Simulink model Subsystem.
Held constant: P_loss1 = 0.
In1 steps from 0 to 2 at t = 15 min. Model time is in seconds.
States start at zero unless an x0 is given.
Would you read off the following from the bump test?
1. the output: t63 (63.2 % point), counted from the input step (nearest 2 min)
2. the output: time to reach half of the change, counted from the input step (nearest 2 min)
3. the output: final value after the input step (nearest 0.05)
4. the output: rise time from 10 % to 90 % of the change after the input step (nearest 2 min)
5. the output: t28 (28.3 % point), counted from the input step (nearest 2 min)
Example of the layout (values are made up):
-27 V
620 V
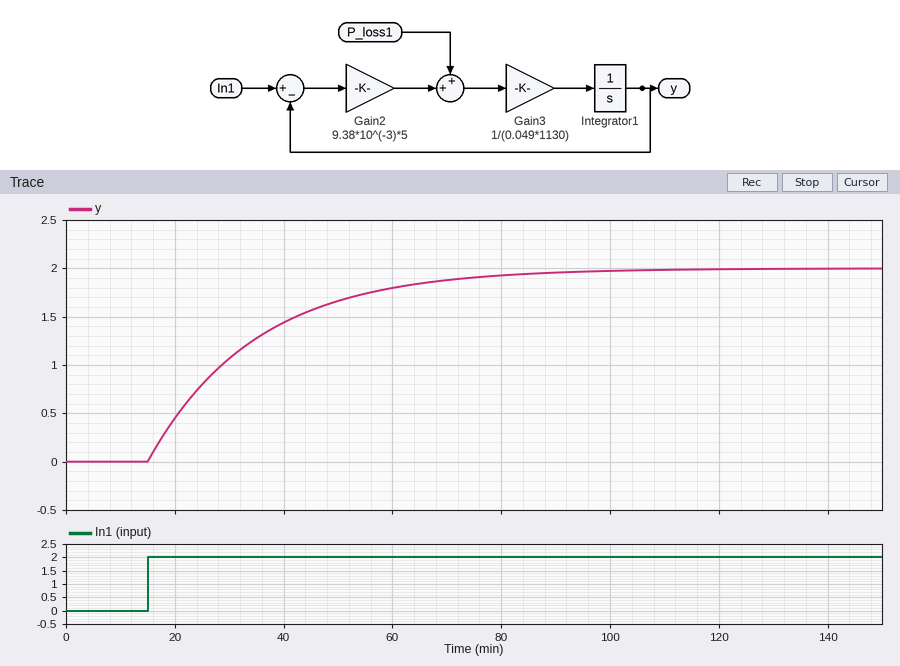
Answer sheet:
20 min
14 min
2.00
44 min
6 min
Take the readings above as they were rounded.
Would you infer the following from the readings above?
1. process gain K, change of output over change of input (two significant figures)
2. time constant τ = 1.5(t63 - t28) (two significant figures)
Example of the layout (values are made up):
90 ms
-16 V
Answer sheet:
1.0
21 min
